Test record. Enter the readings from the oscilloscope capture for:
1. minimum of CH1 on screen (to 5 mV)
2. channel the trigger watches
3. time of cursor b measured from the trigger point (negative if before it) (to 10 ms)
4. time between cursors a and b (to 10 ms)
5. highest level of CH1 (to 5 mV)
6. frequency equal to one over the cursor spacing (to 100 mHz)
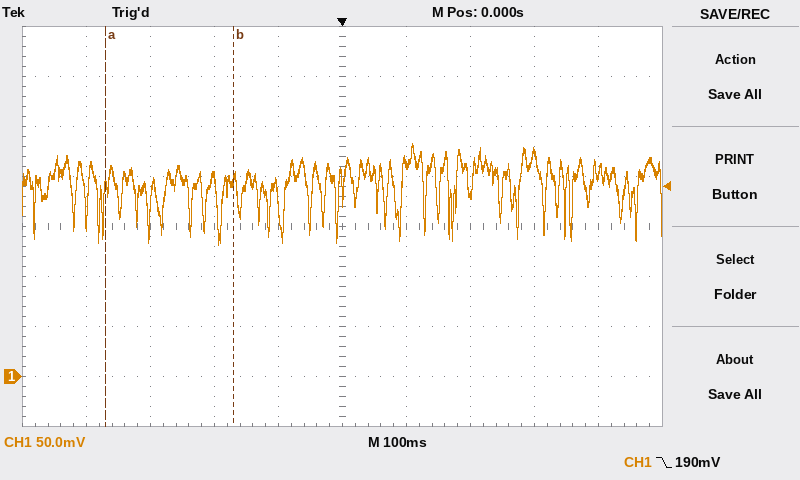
130 mV
CH1
-170 ms
200 ms
235 mV
5.0 Hz
